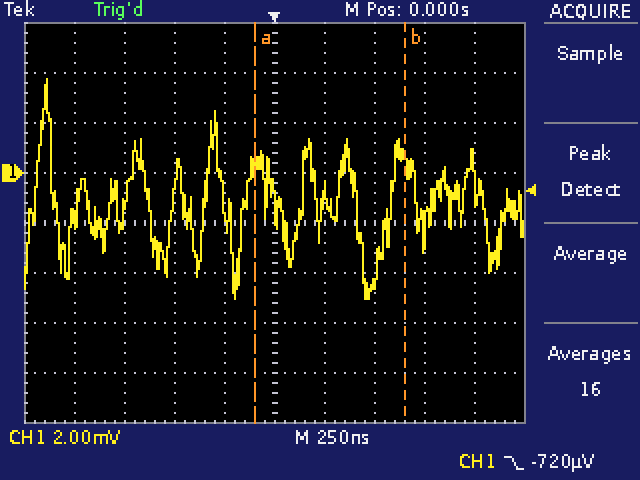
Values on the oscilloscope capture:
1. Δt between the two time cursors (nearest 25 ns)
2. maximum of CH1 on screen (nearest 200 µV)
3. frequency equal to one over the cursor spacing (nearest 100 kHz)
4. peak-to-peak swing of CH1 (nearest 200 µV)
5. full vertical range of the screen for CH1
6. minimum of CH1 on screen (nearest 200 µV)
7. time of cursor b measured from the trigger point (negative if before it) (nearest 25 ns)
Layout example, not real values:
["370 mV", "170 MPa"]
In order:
["750 ns", "3.8 mV", "1.3 MHz", "8.8 mV", "16 mV", "-5.0 mV", "+650 ns"]
